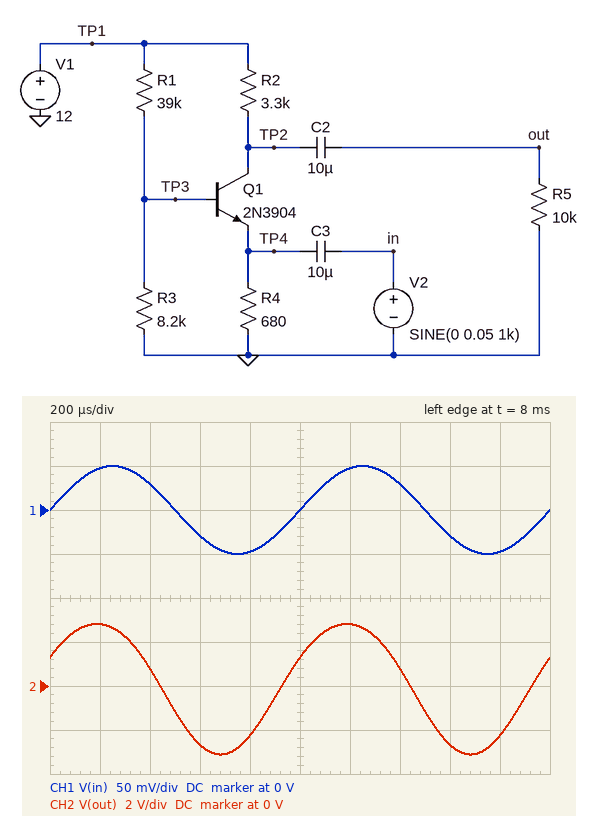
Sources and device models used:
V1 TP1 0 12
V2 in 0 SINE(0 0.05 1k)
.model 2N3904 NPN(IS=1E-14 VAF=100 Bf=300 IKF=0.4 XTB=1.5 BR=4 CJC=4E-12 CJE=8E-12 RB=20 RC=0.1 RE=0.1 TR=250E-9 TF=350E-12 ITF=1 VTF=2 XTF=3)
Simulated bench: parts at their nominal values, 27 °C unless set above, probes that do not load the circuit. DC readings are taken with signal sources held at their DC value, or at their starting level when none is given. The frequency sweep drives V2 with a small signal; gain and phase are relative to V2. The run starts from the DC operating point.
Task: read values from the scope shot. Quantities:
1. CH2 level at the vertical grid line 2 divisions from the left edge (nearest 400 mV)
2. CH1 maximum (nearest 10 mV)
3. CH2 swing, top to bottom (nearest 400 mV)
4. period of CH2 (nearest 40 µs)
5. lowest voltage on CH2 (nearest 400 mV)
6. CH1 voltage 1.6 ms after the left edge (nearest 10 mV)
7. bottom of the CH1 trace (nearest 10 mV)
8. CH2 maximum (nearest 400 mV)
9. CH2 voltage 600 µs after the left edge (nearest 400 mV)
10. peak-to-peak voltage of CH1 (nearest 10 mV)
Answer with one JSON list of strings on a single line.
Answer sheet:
["800 mV", "50 mV", "6.0 V", "1.00 ms", "-3.2 V", "-30 mV", "-50 mV", "2.8 V", "-2.8 V", "100 mV"]
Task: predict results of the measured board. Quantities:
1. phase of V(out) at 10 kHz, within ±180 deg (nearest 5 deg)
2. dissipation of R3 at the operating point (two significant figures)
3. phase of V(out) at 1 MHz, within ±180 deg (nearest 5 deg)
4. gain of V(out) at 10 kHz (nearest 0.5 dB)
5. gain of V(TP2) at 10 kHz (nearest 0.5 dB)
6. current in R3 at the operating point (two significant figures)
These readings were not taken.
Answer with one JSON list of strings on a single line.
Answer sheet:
["0 deg", "510 µW", "-75 deg", "36.5 dB", "36.5 dB", "250 µA"]
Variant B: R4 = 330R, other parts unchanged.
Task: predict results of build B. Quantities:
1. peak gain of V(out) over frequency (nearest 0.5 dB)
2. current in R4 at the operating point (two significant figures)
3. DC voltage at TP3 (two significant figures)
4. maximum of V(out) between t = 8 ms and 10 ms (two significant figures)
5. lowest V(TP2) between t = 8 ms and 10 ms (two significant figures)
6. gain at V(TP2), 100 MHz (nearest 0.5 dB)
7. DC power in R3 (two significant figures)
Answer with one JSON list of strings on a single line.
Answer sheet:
["1.0 dB", "3.3 mA", "1.8 V", "56 mV", "1.1 V", "0 dB", "390 µW"]
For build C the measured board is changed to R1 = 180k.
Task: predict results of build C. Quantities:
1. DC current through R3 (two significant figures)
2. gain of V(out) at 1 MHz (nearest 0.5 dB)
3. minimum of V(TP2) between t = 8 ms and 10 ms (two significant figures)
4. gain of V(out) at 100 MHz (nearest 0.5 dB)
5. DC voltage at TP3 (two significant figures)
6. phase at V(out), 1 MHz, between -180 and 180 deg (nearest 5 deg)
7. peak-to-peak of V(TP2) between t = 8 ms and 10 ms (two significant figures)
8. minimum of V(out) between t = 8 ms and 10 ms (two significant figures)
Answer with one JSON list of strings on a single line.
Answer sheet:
["64 µA", "-7.0 dB", "12 V", "-1.0 dB", "520 mV", "-30 deg", "85 mV", "-72 mV"]
